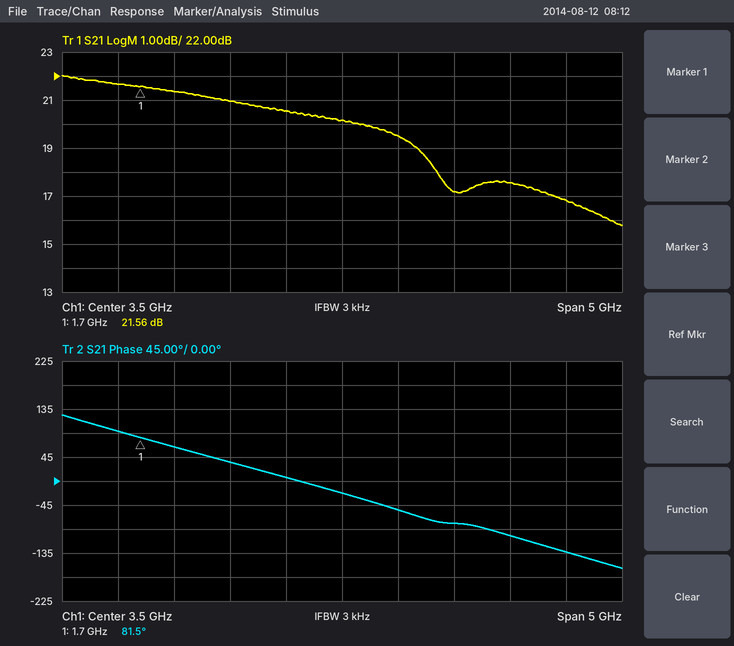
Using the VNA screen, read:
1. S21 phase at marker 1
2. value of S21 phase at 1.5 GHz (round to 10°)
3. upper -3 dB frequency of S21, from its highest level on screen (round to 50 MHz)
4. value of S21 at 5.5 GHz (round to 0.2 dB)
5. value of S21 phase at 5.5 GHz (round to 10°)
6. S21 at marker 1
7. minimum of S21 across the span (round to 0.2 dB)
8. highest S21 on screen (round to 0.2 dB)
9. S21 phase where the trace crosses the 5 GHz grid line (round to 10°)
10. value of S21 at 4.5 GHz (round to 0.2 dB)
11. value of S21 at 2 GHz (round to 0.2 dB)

81.5°
90°
4.15 GHz
16.8 dB
-130°
21.56 dB
15.8 dB
22.0 dB
-100°
17.2 dB
21.4 dB
